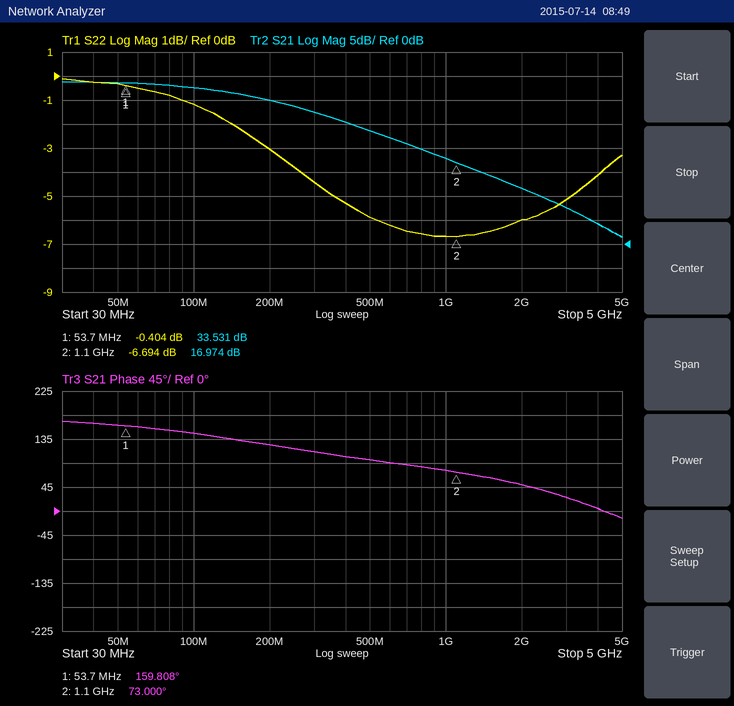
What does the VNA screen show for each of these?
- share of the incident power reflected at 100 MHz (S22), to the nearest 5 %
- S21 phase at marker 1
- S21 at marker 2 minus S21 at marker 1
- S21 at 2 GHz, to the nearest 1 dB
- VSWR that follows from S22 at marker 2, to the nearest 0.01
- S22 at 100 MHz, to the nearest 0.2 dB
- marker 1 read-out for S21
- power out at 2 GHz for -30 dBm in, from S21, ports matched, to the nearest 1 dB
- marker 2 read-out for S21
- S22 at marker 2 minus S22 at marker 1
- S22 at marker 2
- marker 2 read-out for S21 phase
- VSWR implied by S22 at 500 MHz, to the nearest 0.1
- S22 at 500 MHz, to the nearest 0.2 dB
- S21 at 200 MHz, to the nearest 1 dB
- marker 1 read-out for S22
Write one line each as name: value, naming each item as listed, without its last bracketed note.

share of the incident power reflected at 100 MHz (S22), to the nearest 5 %: 75 %
S21 phase at marker 1: 159.808°
S21 at marker 2 minus S21 at marker 1: -16.557 dB
S21 at 2 GHz, to the nearest 1 dB: 12 dB
VSWR that follows from S22 at marker 2, to the nearest 0.01: 2.72
S22 at 100 MHz, to the nearest 0.2 dB: -1.2 dB
marker 1 read-out for S21: 33.531 dB
power out at 2 GHz for -30 dBm in, from S21, ports matched, to the nearest 1 dB: -18 dBm
marker 2 read-out for S21: 16.974 dB
S22 at marker 2 minus S22 at marker 1: -6.290 dB
S22 at marker 2: -6.694 dB
marker 2 read-out for S21 phase: 73.000°
VSWR implied by S22 at 500 MHz, to the nearest 0.1: 3.1
S22 at 500 MHz, to the nearest 0.2 dB: -5.8 dB
S21 at 200 MHz, to the nearest 1 dB: 30 dB
marker 1 read-out for S22: -0.404 dB
